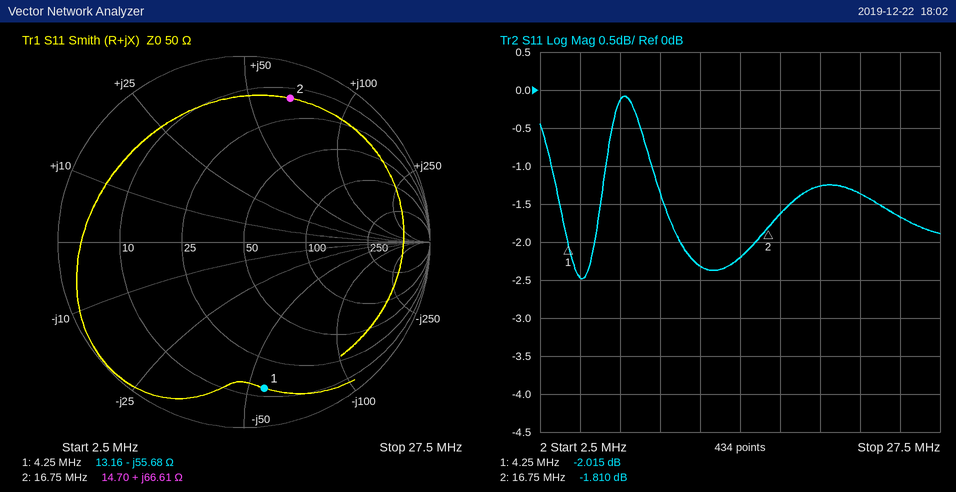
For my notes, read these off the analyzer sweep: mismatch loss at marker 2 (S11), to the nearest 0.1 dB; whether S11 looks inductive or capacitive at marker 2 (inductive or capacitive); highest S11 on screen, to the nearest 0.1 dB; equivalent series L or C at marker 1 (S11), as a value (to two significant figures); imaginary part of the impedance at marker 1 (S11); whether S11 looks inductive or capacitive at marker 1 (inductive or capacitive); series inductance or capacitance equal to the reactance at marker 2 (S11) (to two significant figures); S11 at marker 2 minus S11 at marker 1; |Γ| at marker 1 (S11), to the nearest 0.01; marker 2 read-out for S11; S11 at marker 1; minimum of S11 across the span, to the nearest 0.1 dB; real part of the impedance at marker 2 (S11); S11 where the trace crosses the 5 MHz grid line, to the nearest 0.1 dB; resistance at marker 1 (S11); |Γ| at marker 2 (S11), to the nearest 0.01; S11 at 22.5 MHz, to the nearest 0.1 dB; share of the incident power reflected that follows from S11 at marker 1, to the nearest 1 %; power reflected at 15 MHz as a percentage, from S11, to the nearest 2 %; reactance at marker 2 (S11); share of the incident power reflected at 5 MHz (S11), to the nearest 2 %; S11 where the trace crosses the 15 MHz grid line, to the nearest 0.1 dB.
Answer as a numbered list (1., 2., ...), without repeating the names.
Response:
1. 4.7 dB
2. inductive
3. -0.1 dB
4. 670 pF
5. -55.68 Ω
6. capacitive
7. 630 nH
8. 0.205 dB
9. 0.79
10. -1.810 dB
11. -2.015 dB
12. -2.5 dB
13. 14.70 Ω
14. -2.5 dB
15. 13.16 Ω
16. 0.81
17. -1.4 dB
18. 63 %
19. 60 %
20. +66.61 Ω
21. 56 %
22. -2.2 dB
